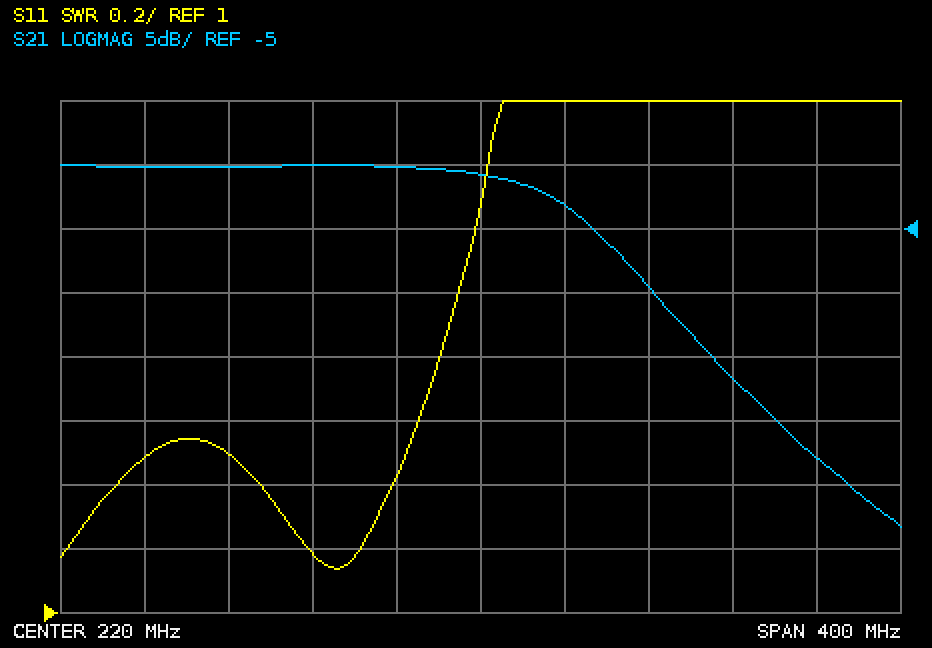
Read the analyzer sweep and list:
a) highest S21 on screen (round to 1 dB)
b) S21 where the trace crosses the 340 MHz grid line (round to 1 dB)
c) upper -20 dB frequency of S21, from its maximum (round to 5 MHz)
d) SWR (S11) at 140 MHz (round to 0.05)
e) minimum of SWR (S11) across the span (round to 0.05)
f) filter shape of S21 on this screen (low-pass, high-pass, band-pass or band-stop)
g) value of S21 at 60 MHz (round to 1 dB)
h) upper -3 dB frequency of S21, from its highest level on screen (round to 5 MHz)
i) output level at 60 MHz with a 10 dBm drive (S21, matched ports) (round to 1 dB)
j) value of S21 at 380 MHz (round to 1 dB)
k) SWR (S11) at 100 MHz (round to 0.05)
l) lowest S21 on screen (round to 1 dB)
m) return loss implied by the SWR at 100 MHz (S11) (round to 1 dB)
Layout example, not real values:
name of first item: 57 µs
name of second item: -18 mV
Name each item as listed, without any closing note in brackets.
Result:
highest S21 on screen: 0 dB
S21 where the trace crosses the 340 MHz grid line: -17 dB
upper -20 dB frequency of S21, from its maximum: 360 MHz
SWR (S11) at 140 MHz: 1.20
minimum of SWR (S11) across the span: 1.15
filter shape of S21 on this screen: low-pass
value of S21 at 60 MHz: 0 dB
upper -3 dB frequency of S21, from its highest level on screen: 260 MHz
output level at 60 MHz with a 10 dBm drive (S21, matched ports): 10 dBm
value of S21 at 380 MHz: -23 dB
SWR (S11) at 100 MHz: 1.50
lowest S21 on screen: -28 dB
return loss implied by the SWR at 100 MHz (S11): 14 dB
